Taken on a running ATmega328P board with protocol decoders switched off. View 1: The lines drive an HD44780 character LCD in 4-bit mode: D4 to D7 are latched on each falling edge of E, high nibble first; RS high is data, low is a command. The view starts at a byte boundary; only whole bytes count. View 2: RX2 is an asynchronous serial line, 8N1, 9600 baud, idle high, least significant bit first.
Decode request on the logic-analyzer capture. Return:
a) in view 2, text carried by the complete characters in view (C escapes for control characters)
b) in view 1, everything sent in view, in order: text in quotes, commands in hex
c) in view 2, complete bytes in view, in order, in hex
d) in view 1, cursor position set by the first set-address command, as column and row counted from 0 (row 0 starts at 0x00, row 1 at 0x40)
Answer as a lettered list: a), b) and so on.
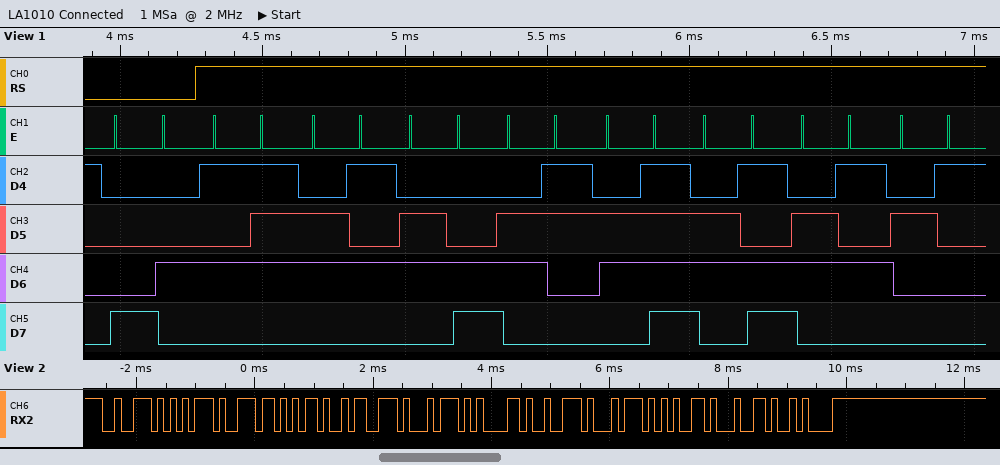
a) "run-started\n"
b) 0x84 "Welcome!"
c) 72 75 6E 2D 73 74 61 72 74 65 64 0A
d) column 4, row 0
